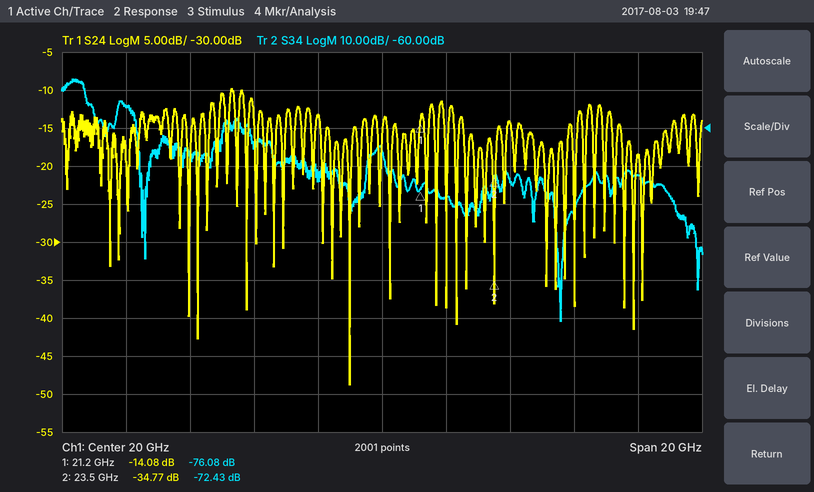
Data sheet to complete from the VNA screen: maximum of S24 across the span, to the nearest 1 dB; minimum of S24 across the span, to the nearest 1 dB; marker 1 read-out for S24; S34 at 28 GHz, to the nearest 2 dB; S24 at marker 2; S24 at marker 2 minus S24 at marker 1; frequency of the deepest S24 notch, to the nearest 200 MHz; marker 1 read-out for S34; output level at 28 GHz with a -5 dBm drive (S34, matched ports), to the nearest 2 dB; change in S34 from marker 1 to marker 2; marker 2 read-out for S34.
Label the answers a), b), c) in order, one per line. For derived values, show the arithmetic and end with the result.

a) -10 dB
b) -49 dB
c) -14.08 dB
d) -72 dB
e) -34.77 dB
f) -34.77 − (-14.08) = -20.69 dB
g) 19.0 GHz
h) -76.08 dB
i) -5 dBm + (-72 dB) = -78 dBm
j) -72.43 − (-76.08) = 3.65 dB
k) -72.43 dB
